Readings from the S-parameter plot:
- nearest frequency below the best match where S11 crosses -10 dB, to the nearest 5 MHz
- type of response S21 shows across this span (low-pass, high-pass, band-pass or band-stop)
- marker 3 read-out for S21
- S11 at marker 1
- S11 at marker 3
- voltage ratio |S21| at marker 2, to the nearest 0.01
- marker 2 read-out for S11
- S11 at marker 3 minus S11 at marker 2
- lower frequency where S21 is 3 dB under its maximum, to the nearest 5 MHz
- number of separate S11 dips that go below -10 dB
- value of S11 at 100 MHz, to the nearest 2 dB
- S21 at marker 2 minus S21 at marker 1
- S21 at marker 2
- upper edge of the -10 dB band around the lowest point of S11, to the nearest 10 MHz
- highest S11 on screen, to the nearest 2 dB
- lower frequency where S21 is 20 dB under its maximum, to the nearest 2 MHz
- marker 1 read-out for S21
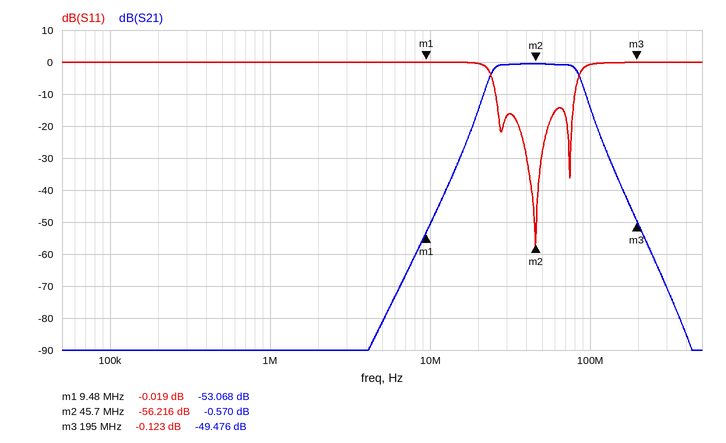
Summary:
25 MHz
band-pass
-49.476 dB
-0.019 dB
-0.123 dB
0.94
-56.216 dB
56.093 dB
25 MHz
3
0 dB
52.498 dB
-0.570 dB
80 MHz
0 dB
18 MHz
-53.068 dB
